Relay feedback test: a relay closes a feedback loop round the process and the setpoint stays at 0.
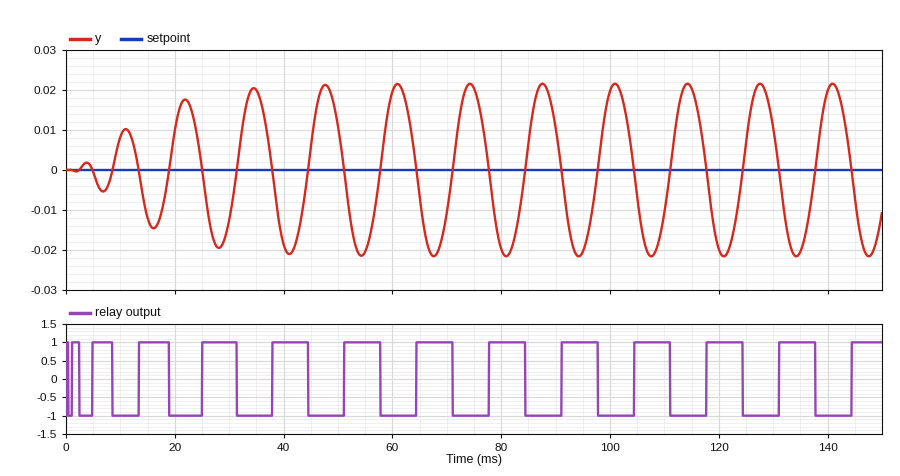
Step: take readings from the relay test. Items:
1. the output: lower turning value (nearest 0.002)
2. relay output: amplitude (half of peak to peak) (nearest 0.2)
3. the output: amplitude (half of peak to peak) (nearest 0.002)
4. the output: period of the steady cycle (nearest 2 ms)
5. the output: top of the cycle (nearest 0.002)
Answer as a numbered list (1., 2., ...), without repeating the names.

1. -0.022
2. 1.0
3. 0.022
4. 14 ms
5. 0.022
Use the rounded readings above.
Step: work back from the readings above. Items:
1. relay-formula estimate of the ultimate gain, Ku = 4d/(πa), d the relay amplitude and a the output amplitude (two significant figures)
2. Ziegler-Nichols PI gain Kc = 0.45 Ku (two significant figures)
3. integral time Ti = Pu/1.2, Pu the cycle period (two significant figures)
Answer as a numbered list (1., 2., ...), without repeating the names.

1. 58
2. 26
3. 12 ms
